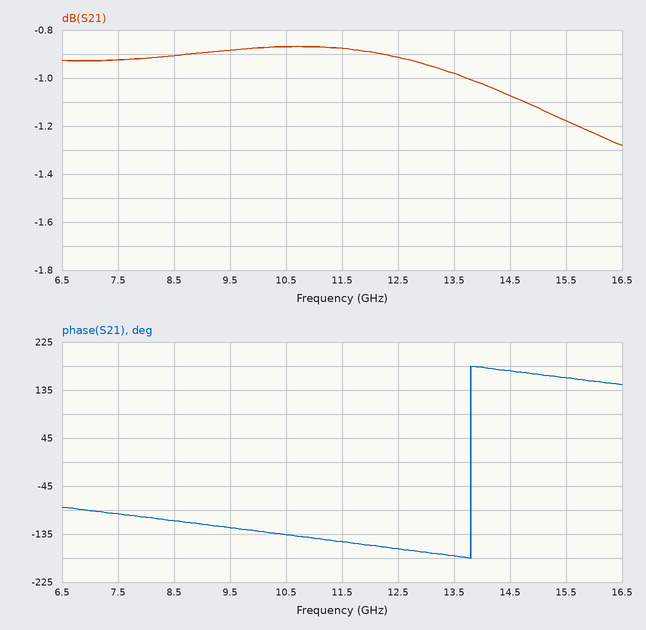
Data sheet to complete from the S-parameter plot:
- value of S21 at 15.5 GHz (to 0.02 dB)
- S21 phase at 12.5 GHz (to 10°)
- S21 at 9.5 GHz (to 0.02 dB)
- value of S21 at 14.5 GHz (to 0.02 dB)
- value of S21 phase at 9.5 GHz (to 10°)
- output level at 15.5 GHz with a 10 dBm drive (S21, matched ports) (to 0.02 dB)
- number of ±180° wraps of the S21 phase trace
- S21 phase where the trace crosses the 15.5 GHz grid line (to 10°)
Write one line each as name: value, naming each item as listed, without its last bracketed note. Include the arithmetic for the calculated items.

value of S21 at 15.5 GHz: -1.18 dB
S21 phase at 12.5 GHz: -160°
S21 at 9.5 GHz: -0.88 dB
value of S21 at 14.5 GHz: -1.08 dB
value of S21 phase at 9.5 GHz: -120°
output level at 15.5 GHz with a 10 dBm drive (S21, matched ports): 10 dBm + (-1.18 dB) = 8.82 dBm
number of ±180° wraps of the S21 phase trace: 1
S21 phase where the trace crosses the 15.5 GHz grid line: 160°
